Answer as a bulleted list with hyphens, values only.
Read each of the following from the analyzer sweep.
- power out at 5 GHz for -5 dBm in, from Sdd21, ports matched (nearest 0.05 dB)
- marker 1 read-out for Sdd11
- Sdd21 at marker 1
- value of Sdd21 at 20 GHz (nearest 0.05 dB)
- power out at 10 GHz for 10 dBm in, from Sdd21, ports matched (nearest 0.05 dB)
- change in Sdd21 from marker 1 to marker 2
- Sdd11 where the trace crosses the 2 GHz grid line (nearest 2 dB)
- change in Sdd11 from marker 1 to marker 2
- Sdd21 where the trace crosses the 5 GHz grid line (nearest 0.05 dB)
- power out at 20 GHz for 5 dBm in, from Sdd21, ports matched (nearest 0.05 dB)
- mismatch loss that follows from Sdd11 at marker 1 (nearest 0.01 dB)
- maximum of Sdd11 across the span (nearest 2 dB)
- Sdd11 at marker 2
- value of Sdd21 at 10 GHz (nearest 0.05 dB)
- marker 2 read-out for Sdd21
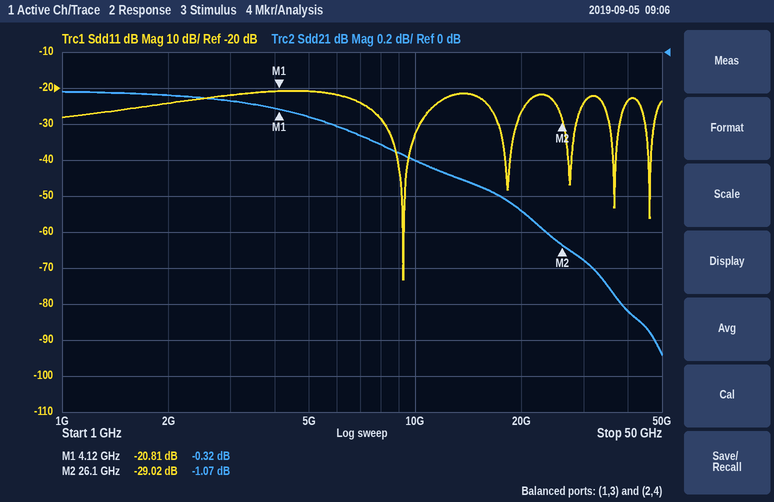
- -5.35 dBm
- -20.81 dB
- -0.32 dB
- -0.90 dB
- 9.40 dBm
- -0.75 dB
- -24 dB
- -8.21 dB
- -0.35 dB
- 4.10 dBm
- 0.04 dB
- -20 dB
- -29.02 dB
- -0.60 dB
- -1.07 dB
